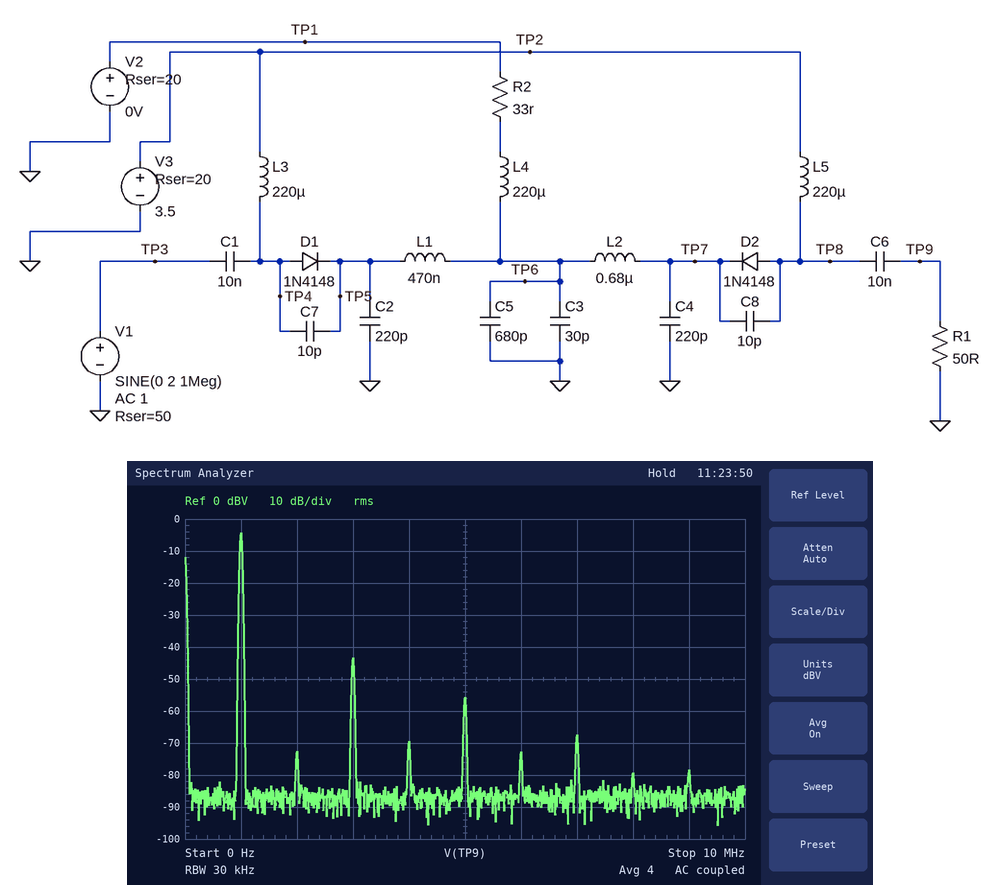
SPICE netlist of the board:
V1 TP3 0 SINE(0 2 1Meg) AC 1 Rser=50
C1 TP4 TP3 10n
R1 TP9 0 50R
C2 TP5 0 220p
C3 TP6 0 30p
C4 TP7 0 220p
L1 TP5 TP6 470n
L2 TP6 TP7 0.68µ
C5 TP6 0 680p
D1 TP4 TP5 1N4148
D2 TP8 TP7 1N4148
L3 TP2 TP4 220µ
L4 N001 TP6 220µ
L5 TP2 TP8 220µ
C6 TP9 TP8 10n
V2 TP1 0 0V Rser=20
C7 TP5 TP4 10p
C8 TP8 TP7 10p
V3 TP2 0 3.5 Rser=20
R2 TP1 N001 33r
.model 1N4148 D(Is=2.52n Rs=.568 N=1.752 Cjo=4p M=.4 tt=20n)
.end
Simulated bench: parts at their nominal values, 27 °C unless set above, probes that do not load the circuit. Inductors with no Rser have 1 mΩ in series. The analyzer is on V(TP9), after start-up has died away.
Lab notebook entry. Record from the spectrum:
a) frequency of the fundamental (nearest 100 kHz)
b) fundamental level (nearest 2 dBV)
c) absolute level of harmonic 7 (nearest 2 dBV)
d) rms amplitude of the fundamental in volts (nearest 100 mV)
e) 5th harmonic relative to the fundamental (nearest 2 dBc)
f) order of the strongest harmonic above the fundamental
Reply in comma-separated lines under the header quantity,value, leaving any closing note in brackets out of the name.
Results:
quantity,value
frequency of the fundamental,1.0 MHz
fundamental level,-4 dBV
absolute level of harmonic 7,-68 dBV
rms amplitude of the fundamental in volts,600 mV
5th harmonic relative to the fundamental,-52 dBc
order of the strongest harmonic above the fundamental,3
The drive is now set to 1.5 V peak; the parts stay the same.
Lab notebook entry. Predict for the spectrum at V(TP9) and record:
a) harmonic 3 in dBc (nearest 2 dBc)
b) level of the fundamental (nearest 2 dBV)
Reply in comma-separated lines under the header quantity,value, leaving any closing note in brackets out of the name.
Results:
quantity,value
harmonic 3 in dBc,-50 dBc
level of the fundamental,-6 dBV
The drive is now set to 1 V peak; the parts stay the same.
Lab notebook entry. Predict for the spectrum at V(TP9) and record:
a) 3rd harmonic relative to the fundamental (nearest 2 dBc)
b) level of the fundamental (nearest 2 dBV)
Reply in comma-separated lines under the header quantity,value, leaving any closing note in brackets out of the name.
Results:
quantity,value
3rd harmonic relative to the fundamental,-58 dBc
level of the fundamental,-10 dBV
